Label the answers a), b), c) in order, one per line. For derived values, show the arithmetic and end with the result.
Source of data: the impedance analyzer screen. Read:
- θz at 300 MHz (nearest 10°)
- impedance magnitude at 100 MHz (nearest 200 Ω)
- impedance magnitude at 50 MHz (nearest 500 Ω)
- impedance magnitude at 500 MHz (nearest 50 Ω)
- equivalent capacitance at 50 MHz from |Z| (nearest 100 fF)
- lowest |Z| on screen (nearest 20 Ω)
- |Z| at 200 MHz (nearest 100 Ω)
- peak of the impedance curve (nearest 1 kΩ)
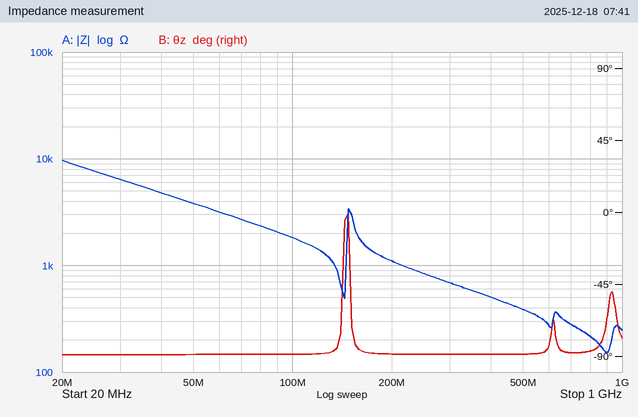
a) -90°
b) 1.8 kΩ
c) 4.0 kΩ
d) 400 Ω
e) C = 1/(2π × 50 MHz × 4.0 kΩ) ≈ 796 fF, so 800 fF to the nearest 100 fF
f) 160 Ω
g) 1.1 kΩ
h) 10 kΩ
